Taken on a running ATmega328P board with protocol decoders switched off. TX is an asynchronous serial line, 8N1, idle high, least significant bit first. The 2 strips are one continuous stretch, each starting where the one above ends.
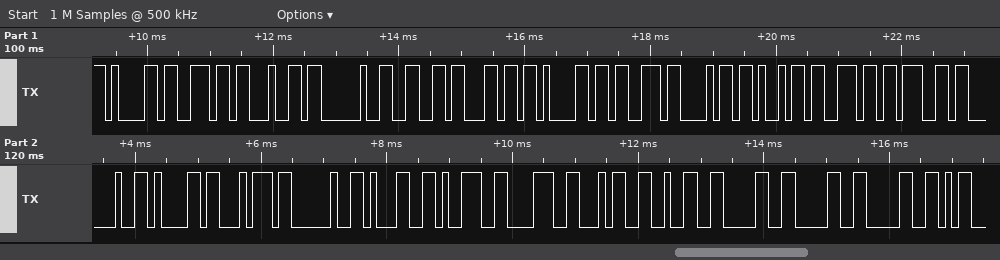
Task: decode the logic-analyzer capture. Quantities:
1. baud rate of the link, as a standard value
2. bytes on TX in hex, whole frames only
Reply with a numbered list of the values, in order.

1. 9600 baud
2. 61 6E 64 20 66 6C 61 73 68 69 6E 67 20 61 74 20 31 39 38 34 32 30 30 30
